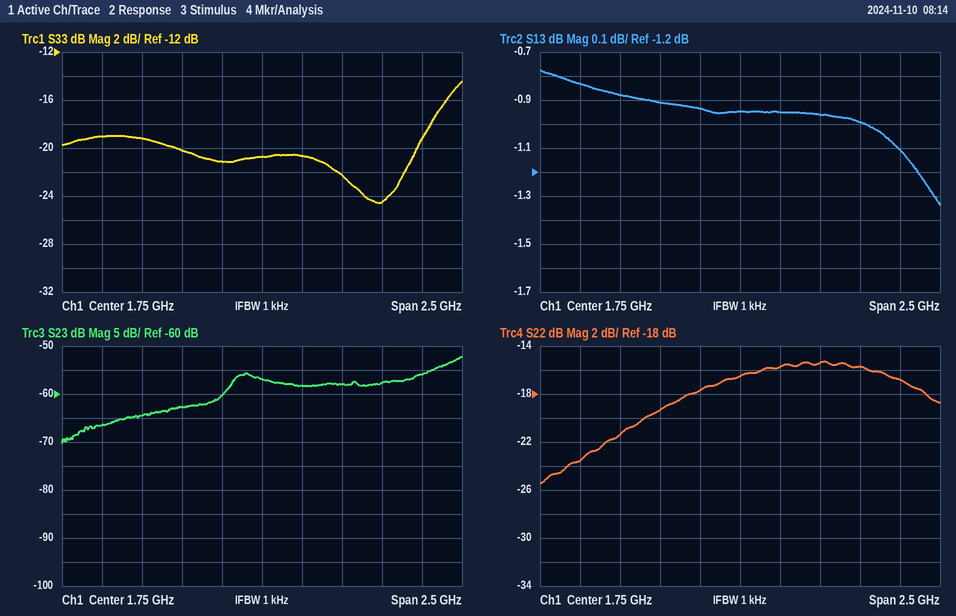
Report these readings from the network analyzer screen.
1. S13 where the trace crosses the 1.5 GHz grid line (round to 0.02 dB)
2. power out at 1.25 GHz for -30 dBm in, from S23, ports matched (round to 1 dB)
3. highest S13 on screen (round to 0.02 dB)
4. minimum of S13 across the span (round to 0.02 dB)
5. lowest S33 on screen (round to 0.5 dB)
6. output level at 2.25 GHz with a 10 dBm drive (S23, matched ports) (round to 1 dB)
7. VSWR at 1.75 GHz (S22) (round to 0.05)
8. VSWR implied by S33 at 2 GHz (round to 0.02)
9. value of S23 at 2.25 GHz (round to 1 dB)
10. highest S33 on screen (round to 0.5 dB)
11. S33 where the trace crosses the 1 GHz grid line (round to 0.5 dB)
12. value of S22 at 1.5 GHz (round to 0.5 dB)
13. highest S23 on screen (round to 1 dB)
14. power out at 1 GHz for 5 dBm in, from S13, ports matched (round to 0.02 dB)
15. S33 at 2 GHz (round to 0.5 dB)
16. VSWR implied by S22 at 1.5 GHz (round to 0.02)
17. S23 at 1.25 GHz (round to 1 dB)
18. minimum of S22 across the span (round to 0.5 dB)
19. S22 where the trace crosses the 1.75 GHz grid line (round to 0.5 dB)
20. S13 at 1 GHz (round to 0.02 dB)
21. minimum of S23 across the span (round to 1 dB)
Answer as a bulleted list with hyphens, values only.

- -0.94 dB
- -93 dBm
- -0.78 dB
- -1.34 dB
- -24.5 dB
- -48 dBm
- 1.35
- 1.20
- -58 dB
- -14.5 dB
- -19.0 dB
- -17.5 dB
- -52 dB
- 4.12 dBm
- -20.5 dB
- 1.30
- -63 dB
- -25.5 dB
- -16.5 dB
- -0.88 dB
- -70 dB
